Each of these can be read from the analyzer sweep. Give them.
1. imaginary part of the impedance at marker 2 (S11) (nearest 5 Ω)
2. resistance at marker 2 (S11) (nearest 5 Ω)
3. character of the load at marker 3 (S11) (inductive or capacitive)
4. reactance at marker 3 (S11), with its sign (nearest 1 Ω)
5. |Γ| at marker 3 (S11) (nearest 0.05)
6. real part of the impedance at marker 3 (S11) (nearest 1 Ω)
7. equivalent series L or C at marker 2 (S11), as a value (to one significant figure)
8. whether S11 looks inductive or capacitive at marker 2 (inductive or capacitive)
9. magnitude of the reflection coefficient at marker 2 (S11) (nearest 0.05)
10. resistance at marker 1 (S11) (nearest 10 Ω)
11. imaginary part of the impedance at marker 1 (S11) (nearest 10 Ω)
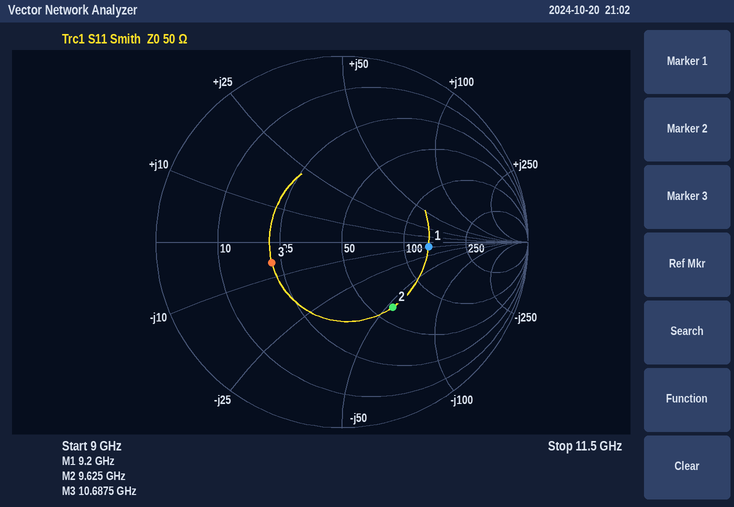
-55 Ω
60 Ω
capacitive
-6 Ω
0.40
22 Ω
300 fF
capacitive
0.45
140 Ω
-10 Ω
